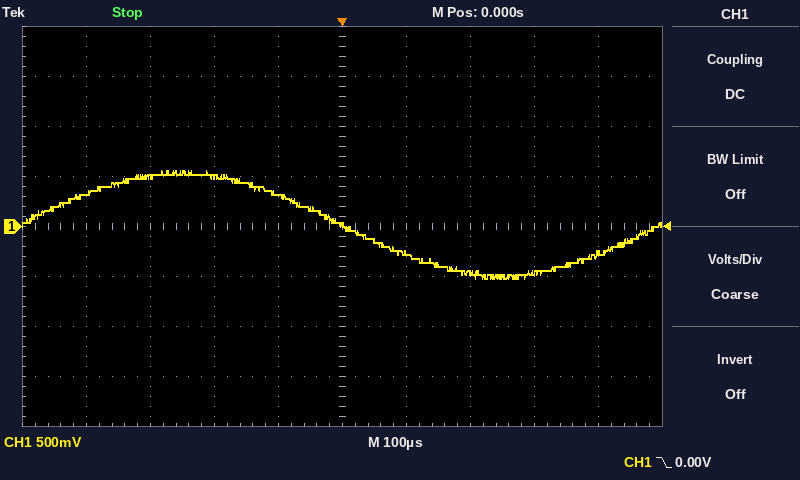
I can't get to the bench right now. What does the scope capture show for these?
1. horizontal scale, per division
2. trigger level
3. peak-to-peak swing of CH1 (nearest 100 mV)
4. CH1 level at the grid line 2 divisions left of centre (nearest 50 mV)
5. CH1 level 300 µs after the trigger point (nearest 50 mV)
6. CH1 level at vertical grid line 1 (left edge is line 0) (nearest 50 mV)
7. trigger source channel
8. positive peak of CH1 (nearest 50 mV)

100 µs
0.00 V
1.10 V
500 mV
-450 mV
350 mV
CH1
550 mV
